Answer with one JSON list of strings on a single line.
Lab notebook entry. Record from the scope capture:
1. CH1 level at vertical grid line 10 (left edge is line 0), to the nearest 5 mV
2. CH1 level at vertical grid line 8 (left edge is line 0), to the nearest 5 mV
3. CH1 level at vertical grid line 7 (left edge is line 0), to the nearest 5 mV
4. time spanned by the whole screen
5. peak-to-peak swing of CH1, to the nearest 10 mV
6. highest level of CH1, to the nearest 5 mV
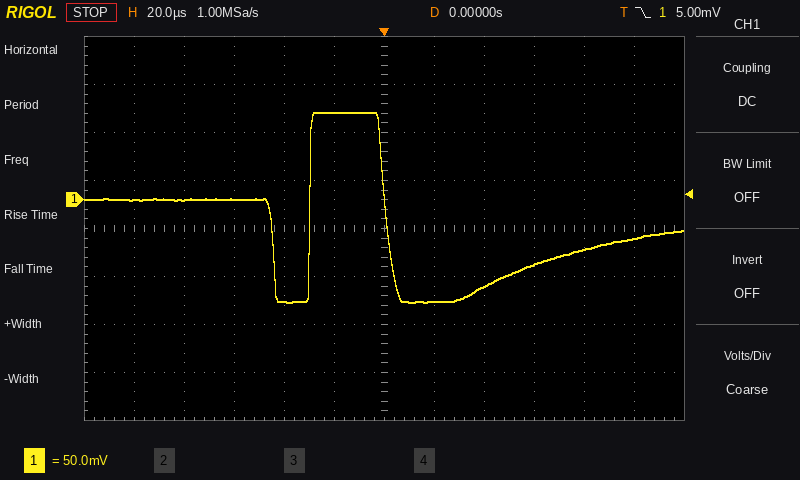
["-50 mV", "-90 mV", "-105 mV", "240 µs", "200 mV", "90 mV"]
